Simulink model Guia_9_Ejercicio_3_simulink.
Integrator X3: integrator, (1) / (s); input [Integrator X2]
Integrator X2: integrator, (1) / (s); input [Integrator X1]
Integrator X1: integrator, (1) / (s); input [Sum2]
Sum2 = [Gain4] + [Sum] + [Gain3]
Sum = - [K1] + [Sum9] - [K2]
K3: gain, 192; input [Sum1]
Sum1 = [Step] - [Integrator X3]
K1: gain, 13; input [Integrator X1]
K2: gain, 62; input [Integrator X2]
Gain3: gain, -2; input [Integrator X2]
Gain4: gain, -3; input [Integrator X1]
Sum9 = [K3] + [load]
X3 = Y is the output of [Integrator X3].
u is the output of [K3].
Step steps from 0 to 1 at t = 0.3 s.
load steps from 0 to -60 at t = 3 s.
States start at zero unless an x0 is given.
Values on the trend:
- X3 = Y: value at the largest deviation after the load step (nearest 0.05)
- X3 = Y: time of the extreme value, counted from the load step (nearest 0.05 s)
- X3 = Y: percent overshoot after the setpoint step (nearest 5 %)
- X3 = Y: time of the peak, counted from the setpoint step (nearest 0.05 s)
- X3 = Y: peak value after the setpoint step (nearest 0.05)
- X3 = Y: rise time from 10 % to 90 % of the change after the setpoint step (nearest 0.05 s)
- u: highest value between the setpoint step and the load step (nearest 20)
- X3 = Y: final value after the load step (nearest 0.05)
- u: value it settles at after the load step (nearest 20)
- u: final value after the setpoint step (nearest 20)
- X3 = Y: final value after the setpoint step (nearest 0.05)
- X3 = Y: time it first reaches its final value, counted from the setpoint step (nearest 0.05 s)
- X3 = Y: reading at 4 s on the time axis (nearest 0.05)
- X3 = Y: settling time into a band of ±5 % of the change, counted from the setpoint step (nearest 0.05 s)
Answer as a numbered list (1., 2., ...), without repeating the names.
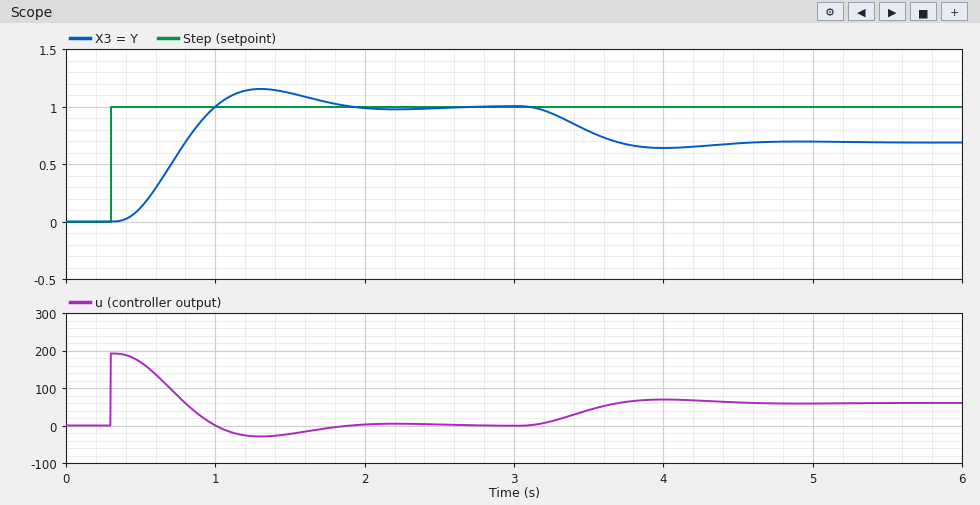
1. 0.65
2. 1.00 s
3. 15 %
4. 1.00 s
5. 1.15
6. 0.45 s
7. 200
8. 0.70
9. 60
10. 0
11. 1.00
12. 0.70 s
13. 0.65
14. 1.40 s
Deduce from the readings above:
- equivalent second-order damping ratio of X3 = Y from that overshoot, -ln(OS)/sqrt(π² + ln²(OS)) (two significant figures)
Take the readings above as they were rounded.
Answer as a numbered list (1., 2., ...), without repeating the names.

1. 0.52
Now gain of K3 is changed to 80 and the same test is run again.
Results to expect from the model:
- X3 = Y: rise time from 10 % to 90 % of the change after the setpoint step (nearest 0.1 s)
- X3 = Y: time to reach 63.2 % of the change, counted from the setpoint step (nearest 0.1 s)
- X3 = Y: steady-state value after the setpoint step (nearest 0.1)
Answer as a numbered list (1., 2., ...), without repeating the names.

1. 1.2 s
2. 0.9 s
3. 1.0
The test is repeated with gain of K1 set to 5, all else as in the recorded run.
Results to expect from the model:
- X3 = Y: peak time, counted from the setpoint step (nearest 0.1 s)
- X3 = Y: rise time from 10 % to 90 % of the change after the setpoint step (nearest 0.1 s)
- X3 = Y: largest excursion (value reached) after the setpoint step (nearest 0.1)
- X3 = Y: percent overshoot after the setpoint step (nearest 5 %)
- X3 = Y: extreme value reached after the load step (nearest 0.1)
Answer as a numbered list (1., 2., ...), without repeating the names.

1. 0.7 s
2. 0.3 s
3. 1.1
4. 10 %
5. 0.7
